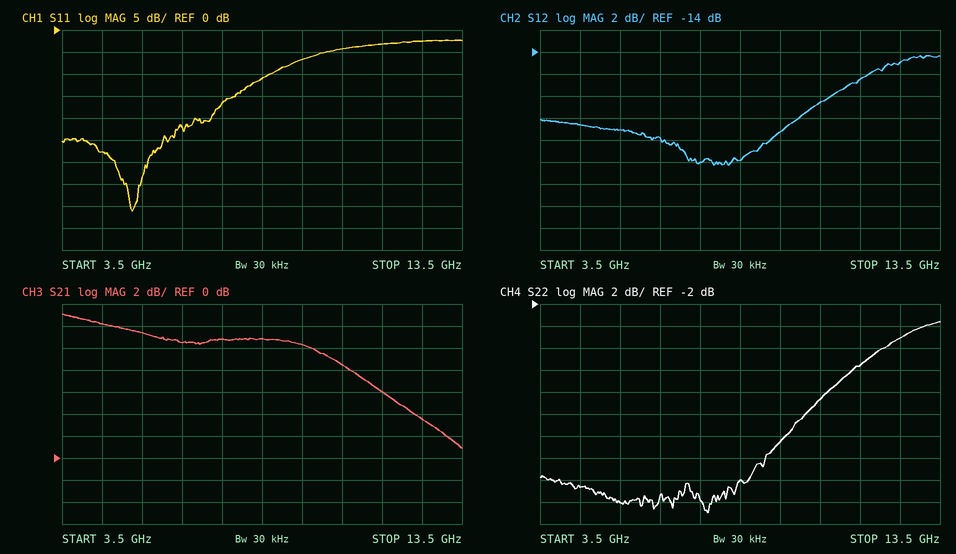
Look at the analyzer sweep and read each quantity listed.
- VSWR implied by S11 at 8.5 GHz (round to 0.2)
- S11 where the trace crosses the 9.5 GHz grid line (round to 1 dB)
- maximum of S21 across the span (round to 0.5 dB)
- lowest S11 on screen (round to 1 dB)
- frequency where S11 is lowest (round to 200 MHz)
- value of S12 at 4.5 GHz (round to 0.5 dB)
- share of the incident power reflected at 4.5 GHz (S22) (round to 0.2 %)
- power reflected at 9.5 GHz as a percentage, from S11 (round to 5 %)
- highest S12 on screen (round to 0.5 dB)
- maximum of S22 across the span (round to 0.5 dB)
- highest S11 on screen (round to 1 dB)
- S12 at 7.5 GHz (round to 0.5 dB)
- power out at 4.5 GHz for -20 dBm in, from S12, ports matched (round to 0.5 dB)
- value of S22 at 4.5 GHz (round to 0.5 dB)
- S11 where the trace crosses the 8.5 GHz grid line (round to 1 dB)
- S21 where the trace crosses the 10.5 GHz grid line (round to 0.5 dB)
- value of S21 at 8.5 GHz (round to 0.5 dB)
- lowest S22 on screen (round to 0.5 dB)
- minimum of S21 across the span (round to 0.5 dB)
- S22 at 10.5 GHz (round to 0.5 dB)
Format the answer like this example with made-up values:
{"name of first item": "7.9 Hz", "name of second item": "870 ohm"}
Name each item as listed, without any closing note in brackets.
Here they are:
{"VSWR implied by S11 at 8.5 GHz": "1.8", "S11 where the trace crosses the 9.5 GHz grid line": "-7 dB", "maximum of S21 across the span": "13.0 dB", "lowest S11 on screen": "-41 dB", "frequency where S11 is lowest": "5.2 GHz", "value of S12 at 4.5 GHz": "-20.5 dB", "share of the incident power reflected at 4.5 GHz (S22)": "1.4 %", "power reflected at 9.5 GHz as a percentage, from S11": "20 %", "highest S12 on screen": "-14.5 dB", "maximum of S22 across the span": "-3.5 dB", "highest S11 on screen": "-2 dB", "S12 at 7.5 GHz": "-24.0 dB", "power out at 4.5 GHz for -20 dBm in, from S12, ports matched": "-40.5 dBm", "value of S22 at 4.5 GHz": "-18.5 dB", "S11 where the trace crosses the 8.5 GHz grid line": "-11 dB", "S21 where the trace crosses the 10.5 GHz grid line": "8.5 dB", "value of S21 at 8.5 GHz": "11.0 dB", "lowest S22 on screen": "-21.0 dB", "minimum of S21 across the span": "1.0 dB", "S22 at 10.5 GHz": "-10.5 dB"}
